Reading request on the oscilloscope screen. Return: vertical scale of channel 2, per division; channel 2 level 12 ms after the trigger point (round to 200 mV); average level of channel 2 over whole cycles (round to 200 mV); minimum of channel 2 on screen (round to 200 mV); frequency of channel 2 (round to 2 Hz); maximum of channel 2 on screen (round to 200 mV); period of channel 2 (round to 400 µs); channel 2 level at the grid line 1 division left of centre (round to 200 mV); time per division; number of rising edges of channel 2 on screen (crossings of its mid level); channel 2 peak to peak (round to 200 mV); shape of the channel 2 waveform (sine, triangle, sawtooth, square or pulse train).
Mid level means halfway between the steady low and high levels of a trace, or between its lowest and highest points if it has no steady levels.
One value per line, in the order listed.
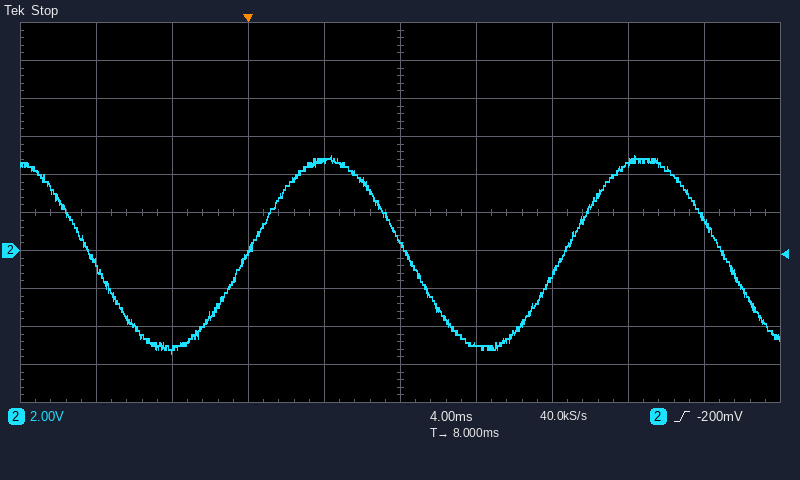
2 V
-5.0 V
-200 mV
-5.4 V
60 Hz
5.0 V
16.8 ms
4.8 V
4 ms
2
10.4 V
sine
